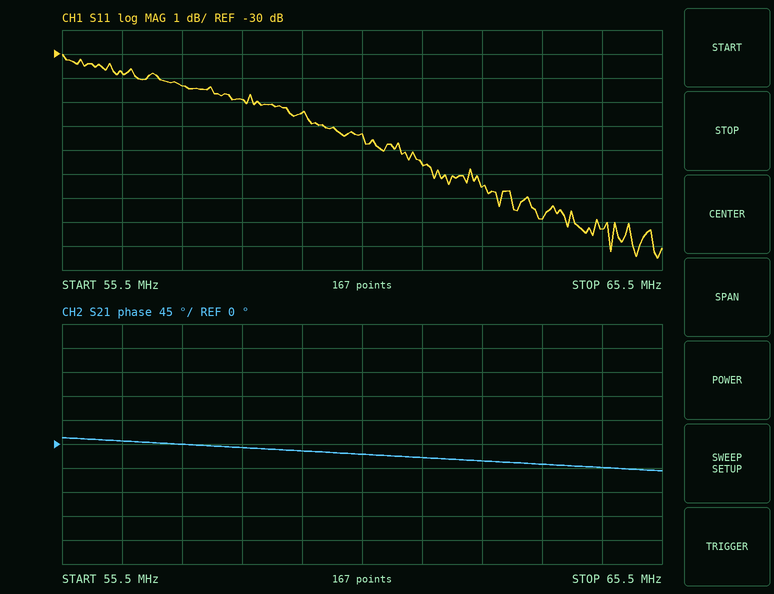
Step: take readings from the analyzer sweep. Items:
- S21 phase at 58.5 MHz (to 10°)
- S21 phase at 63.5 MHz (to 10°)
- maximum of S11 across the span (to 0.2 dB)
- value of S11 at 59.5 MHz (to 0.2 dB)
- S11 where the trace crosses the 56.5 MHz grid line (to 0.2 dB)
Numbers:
-10°
-40°
-30.0 dB
-32.4 dB
-30.8 dB
